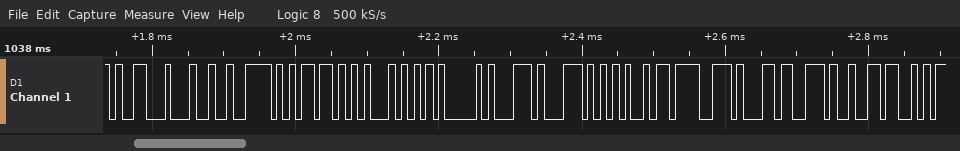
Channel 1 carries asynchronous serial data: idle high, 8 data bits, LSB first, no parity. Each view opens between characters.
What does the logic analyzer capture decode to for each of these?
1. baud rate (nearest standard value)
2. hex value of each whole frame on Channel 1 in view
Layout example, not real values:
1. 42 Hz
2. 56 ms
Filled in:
1. 115200 baud
2. 19, 24, 5E, 5B, 51, 05, 71, 5C, A5, CF, B1, 2E, 36
